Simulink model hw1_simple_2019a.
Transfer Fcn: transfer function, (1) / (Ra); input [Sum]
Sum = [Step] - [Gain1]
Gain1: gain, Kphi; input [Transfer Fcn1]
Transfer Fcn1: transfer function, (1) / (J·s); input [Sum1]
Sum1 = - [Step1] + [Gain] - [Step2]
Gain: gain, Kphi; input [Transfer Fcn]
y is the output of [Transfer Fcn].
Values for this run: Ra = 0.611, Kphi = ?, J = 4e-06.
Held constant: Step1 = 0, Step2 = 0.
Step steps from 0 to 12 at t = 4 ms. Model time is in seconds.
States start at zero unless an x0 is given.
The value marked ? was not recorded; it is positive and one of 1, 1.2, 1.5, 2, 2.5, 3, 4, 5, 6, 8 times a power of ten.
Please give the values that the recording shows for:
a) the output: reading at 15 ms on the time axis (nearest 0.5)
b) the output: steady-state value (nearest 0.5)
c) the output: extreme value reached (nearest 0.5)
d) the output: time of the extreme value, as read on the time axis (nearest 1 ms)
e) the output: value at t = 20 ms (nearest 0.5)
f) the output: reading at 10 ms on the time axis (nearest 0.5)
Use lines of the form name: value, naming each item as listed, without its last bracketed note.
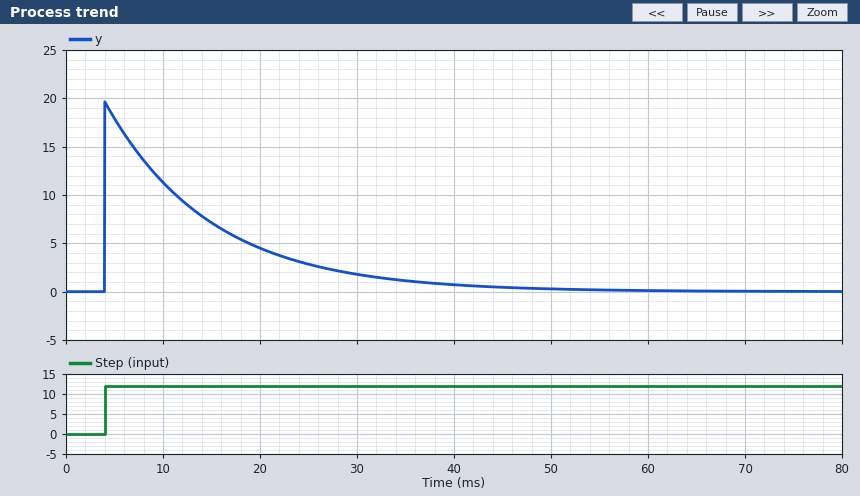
the output: reading at 15 ms on the time axis: 7.0
the output: steady-state value: 0.0
the output: extreme value reached: 19.5
the output: time of the extreme value, as read on the time axis: 4 ms
the output: value at t = 20 ms: 4.5
the output: reading at 10 ms on the time axis: 11.5
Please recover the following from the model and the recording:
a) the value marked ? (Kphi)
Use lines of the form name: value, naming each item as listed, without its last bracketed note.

the value marked ?: 0.015
